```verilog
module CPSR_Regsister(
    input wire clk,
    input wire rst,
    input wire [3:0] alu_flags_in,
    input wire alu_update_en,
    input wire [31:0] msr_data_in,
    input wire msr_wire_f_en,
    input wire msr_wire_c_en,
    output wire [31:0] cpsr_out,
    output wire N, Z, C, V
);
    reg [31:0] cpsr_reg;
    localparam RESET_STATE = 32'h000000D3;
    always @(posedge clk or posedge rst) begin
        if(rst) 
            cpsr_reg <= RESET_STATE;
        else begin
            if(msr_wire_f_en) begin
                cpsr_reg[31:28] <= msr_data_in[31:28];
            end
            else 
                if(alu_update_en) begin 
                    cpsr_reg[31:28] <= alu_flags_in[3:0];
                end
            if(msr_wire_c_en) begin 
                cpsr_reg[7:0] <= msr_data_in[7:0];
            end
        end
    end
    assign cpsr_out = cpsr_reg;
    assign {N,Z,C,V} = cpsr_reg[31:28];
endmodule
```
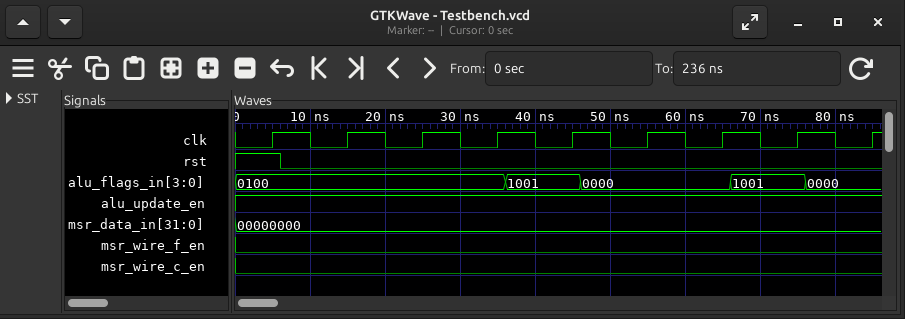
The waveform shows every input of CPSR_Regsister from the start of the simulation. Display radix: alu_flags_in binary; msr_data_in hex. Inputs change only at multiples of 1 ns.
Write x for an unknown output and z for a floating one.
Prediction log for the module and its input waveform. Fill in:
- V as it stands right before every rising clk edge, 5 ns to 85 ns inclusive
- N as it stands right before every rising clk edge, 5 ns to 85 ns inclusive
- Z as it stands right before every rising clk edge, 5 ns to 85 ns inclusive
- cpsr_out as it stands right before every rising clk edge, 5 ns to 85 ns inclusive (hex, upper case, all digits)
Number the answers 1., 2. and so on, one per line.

1. 0 0 0 0 0 1 0 0 1
2. 0 0 0 0 0 1 0 0 1
3. 0 0 1 1 1 0 0 0 0
4. 000000D3, 000000D3, 400000D3, 400000D3, 400000D3, 900000D3, 000000D3, 000000D3, 900000D3
